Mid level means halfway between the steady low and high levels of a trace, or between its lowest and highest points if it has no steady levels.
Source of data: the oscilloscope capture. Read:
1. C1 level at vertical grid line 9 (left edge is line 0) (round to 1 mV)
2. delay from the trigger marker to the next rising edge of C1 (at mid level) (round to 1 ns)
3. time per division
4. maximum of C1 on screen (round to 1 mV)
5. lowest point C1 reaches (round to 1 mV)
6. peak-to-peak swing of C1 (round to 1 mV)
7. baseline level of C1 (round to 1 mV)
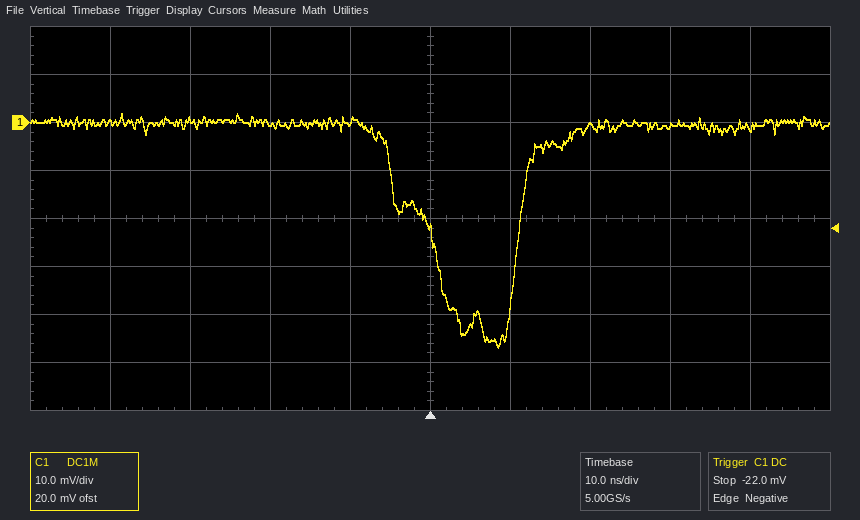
-1 mV
11 ns
10 ns
2 mV
-47 mV
49 mV
0 mV
